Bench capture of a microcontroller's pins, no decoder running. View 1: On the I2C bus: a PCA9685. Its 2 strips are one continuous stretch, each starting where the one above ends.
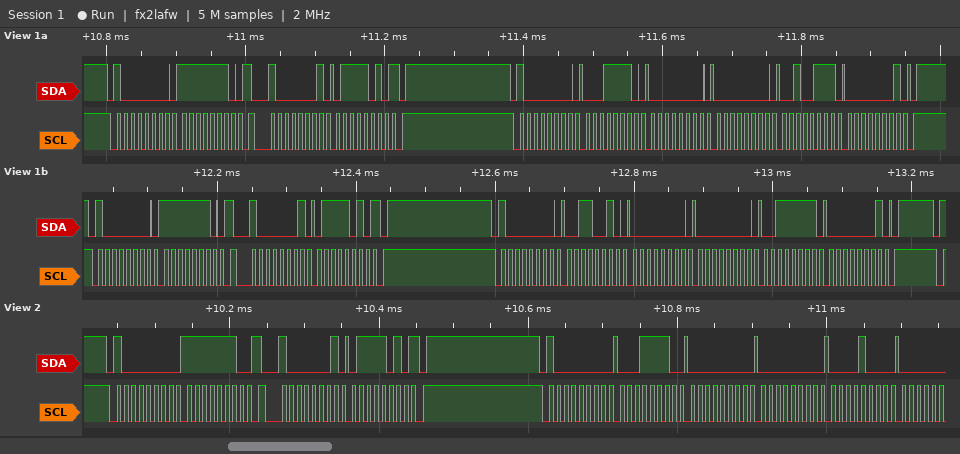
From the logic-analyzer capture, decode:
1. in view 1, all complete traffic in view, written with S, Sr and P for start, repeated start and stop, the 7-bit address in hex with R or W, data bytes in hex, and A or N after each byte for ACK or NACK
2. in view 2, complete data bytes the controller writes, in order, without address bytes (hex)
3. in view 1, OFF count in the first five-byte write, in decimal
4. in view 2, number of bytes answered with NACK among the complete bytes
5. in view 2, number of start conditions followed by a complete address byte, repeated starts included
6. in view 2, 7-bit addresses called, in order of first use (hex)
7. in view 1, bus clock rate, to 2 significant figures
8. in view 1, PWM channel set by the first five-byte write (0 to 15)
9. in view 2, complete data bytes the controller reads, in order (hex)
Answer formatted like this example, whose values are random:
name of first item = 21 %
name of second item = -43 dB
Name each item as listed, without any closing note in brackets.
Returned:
in view 1, all complete traffic in view, written with S, Sr and P for start, repeated start and stop, the 7-bit address in hex with R or W, data bytes in hex, and A or N after each byte for ACK or NACK = S 40W A FE A Sr 40R A 7A N P S 40W A 1E A 00 A 00 A 27 A 01 A P S 40W A FE A Sr 40R A 7A N P S 40W A 32 A 00 A 00 A 3F A 01 A P
in view 2, complete data bytes the controller writes, in order, without address bytes = FE 1E 00 00 08
in view 1, OFF count in the first five-byte write, in decimal = 295
in view 2, number of bytes answered with NACK among the complete bytes = 1
in view 2, number of start conditions followed by a complete address byte, repeated starts included = 3
in view 2, 7-bit addresses called, in order of first use = 0x40
in view 1, bus clock rate, to 2 significant figures = 100 kHz
in view 1, PWM channel set by the first five-byte write = 6
in view 2, complete data bytes the controller reads, in order = 7A
